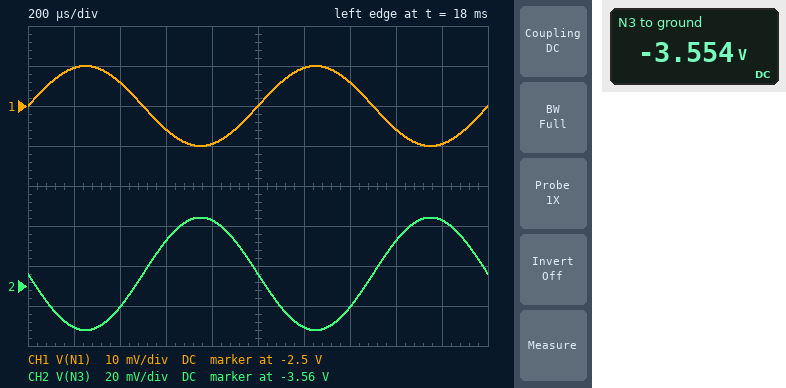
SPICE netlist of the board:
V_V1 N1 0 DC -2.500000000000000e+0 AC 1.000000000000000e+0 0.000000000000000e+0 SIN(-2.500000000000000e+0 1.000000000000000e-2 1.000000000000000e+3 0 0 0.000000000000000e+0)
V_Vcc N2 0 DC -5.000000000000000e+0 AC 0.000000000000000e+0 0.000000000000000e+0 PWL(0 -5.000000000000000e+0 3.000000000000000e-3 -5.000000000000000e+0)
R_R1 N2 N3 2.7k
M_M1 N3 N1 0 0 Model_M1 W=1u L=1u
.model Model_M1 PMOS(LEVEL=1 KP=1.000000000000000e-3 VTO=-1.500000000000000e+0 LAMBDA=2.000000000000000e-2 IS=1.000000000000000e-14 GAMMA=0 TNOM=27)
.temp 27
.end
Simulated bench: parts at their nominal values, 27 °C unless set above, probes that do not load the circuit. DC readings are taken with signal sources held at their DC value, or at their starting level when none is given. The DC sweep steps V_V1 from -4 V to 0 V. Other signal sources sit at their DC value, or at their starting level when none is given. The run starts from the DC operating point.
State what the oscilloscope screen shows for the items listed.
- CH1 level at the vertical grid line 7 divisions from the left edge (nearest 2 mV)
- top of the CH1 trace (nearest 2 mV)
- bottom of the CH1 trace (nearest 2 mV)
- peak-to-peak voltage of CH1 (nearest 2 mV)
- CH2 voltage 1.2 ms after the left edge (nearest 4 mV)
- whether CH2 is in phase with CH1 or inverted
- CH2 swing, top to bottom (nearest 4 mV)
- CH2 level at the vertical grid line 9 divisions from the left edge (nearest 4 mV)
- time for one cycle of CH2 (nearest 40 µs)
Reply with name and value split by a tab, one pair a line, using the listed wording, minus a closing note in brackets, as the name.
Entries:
CH1 level at the vertical grid line 7 divisions from the left edge	-2.494 V
top of the CH1 trace	-2.490 V
bottom of the CH1 trace	-2.510 V
peak-to-peak voltage of CH1	20 mV
CH2 voltage 1.2 ms after the left edge	-3.580 V
whether CH2 is in phase with CH1 or inverted	inverted
CH2 swing, top to bottom	56 mV
CH2 level at the vertical grid line 9 divisions from the left edge	-3.528 V
time for one cycle of CH2	1.00 ms
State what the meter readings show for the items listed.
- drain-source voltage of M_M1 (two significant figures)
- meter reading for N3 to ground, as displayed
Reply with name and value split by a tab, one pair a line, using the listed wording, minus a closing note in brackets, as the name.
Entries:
drain-source voltage of M_M1	-3.6 V
meter reading for N3 to ground, as displayed	-3.554 V
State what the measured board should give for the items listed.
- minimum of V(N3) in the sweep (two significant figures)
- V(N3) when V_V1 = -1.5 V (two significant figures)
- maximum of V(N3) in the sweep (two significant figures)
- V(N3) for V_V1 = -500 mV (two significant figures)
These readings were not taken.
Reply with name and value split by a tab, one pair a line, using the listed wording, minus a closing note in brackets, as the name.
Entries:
minimum of V(N3) in the sweep	-5.0 V
V(N3) when V_V1 = -1.5 V	-5.0 V
maximum of V(N3) in the sweep	-730 mV
V(N3) for V_V1 = -500 mV	-5.0 V
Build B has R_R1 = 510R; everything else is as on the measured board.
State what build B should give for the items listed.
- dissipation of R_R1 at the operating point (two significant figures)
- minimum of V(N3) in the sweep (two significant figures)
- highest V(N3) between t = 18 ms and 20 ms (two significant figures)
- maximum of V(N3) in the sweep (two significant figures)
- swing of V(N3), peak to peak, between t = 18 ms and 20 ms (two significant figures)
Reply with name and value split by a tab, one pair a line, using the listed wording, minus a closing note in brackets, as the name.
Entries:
dissipation of R_R1 at the operating point	150 µW
minimum of V(N3) in the sweep	-5.0 V
highest V(N3) between t = 18 ms and 20 ms	-4.7 V
maximum of V(N3) in the sweep	-3.3 V
swing of V(N3), peak to peak, between t = 18 ms and 20 ms	11 mV
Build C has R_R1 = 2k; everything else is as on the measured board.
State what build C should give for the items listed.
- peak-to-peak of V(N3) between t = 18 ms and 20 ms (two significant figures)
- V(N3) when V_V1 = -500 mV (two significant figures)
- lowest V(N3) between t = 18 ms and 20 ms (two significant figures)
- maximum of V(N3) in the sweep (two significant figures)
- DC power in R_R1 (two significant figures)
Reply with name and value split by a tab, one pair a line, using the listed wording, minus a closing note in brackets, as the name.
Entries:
peak-to-peak of V(N3) between t = 18 ms and 20 ms	42 mV
V(N3) when V_V1 = -500 mV	-5.0 V
lowest V(N3) between t = 18 ms and 20 ms	-3.9 V
maximum of V(N3) in the sweep	-980 mV
DC power in R_R1	580 µW
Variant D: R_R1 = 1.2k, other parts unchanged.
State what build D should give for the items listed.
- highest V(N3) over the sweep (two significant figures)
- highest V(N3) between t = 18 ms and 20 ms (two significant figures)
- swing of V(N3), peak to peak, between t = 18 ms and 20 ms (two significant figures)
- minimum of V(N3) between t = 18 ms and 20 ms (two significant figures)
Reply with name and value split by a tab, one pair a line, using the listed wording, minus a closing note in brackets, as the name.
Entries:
highest V(N3) over the sweep	-1.6 V
highest V(N3) between t = 18 ms and 20 ms	-4.3 V
swing of V(N3), peak to peak, between t = 18 ms and 20 ms	26 mV
minimum of V(N3) between t = 18 ms and 20 ms	-4.4 V
